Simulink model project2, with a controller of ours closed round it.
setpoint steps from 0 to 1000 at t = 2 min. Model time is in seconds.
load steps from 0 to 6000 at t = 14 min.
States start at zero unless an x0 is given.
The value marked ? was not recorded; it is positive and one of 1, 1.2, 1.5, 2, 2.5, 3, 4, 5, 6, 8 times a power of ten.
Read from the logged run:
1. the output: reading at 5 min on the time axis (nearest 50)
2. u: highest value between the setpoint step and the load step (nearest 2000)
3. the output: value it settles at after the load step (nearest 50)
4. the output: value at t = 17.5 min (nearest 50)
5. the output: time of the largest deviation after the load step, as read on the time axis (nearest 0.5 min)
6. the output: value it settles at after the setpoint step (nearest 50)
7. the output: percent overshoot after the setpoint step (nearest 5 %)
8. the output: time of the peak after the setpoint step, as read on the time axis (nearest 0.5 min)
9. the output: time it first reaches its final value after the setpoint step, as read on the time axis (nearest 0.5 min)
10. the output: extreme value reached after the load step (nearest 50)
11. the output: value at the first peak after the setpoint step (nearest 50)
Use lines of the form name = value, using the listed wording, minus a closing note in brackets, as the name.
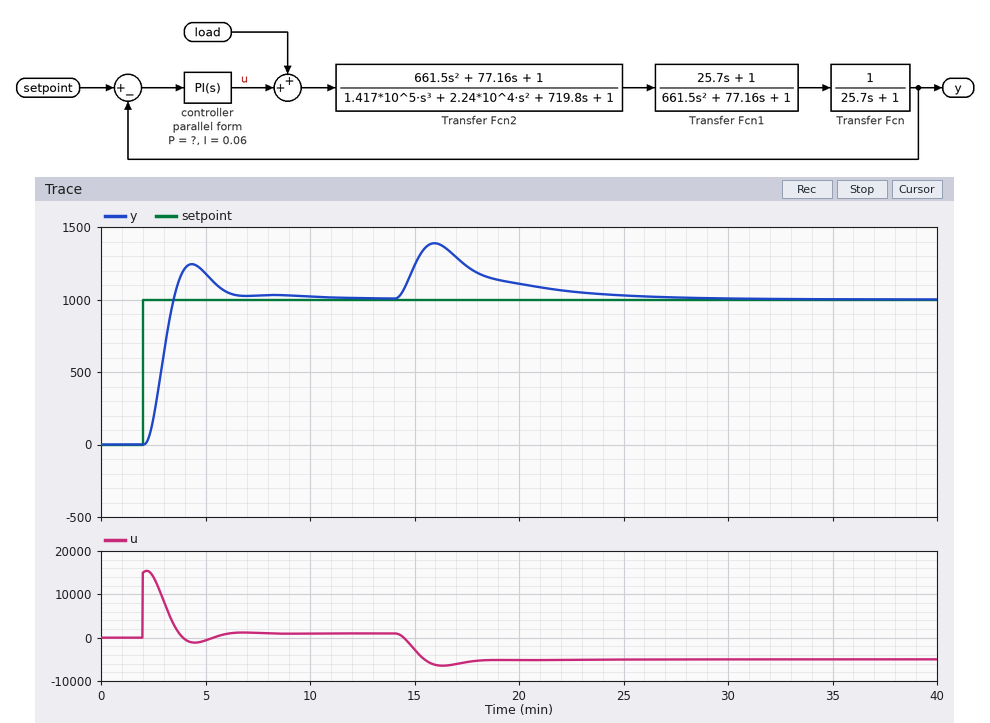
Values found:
the output: reading at 5 min on the time axis = 1200
u: highest value between the setpoint step and the load step = 16000
the output: value it settles at after the load step = 1000
the output: value at t = 17.5 min = 1250
the output: time of the largest deviation after the load step, as read on the time axis = 16.0 min
the output: value it settles at after the setpoint step = 1000
the output: percent overshoot after the setpoint step = 25 %
the output: time of the peak after the setpoint step, as read on the time axis = 4.5 min
the output: time it first reaches its final value after the setpoint step, as read on the time axis = 3.5 min
the output: extreme value reached after the load step = 1400
the output: value at the first peak after the setpoint step = 1250
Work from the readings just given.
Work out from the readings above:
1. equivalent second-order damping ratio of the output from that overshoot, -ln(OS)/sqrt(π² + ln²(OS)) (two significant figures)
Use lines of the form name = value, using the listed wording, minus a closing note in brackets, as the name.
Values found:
equivalent second-order damping ratio of the output from that overshoot, -ln(OS)/sqrt(π² + ln²(OS)) = 0.40
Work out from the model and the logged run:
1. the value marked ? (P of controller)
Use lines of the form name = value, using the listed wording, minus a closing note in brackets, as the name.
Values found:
the value marked ? = 15
